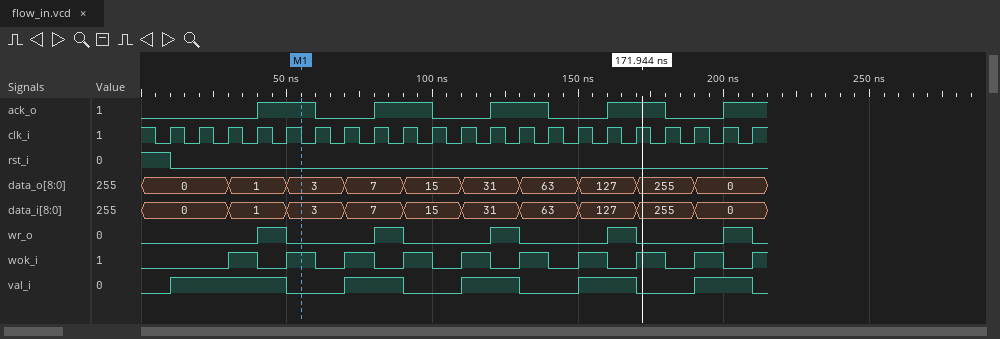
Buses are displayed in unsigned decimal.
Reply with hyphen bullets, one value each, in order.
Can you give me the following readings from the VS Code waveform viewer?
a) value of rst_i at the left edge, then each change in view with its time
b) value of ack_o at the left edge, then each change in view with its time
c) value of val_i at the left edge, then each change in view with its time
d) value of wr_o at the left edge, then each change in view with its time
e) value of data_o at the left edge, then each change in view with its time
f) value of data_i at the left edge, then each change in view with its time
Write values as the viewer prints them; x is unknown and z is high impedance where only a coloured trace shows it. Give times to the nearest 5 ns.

- 1, 0 at 10 ns
- 0, 1 at 40 ns, 0 at 60 ns, 1 at 80 ns, 0 at 100 ns, 1 at 120 ns, 0 at 140 ns, 1 at 160 ns, 0 at 180 ns, 1 at 200 ns
- 0, 1 at 10 ns, 0 at 50 ns, 1 at 70 ns, 0 at 90 ns, 1 at 110 ns, 0 at 130 ns, 1 at 150 ns, 0 at 170 ns, 1 at 190 ns, 0 at 210 ns
- 0, 1 at 40 ns, 0 at 50 ns, 1 at 80 ns, 0 at 90 ns, 1 at 120 ns, 0 at 130 ns, 1 at 160 ns, 0 at 170 ns, 1 at 200 ns, 0 at 210 ns
- 0, 1 at 30 ns, 3 at 50 ns, 7 at 70 ns, 15 at 90 ns, 31 at 110 ns, 63 at 130 ns, 127 at 150 ns, 255 at 170 ns, 0 at 190 ns
- 0, 1 at 30 ns, 3 at 50 ns, 7 at 70 ns, 15 at 90 ns, 31 at 110 ns, 63 at 130 ns, 127 at 150 ns, 255 at 170 ns, 0 at 190 ns
